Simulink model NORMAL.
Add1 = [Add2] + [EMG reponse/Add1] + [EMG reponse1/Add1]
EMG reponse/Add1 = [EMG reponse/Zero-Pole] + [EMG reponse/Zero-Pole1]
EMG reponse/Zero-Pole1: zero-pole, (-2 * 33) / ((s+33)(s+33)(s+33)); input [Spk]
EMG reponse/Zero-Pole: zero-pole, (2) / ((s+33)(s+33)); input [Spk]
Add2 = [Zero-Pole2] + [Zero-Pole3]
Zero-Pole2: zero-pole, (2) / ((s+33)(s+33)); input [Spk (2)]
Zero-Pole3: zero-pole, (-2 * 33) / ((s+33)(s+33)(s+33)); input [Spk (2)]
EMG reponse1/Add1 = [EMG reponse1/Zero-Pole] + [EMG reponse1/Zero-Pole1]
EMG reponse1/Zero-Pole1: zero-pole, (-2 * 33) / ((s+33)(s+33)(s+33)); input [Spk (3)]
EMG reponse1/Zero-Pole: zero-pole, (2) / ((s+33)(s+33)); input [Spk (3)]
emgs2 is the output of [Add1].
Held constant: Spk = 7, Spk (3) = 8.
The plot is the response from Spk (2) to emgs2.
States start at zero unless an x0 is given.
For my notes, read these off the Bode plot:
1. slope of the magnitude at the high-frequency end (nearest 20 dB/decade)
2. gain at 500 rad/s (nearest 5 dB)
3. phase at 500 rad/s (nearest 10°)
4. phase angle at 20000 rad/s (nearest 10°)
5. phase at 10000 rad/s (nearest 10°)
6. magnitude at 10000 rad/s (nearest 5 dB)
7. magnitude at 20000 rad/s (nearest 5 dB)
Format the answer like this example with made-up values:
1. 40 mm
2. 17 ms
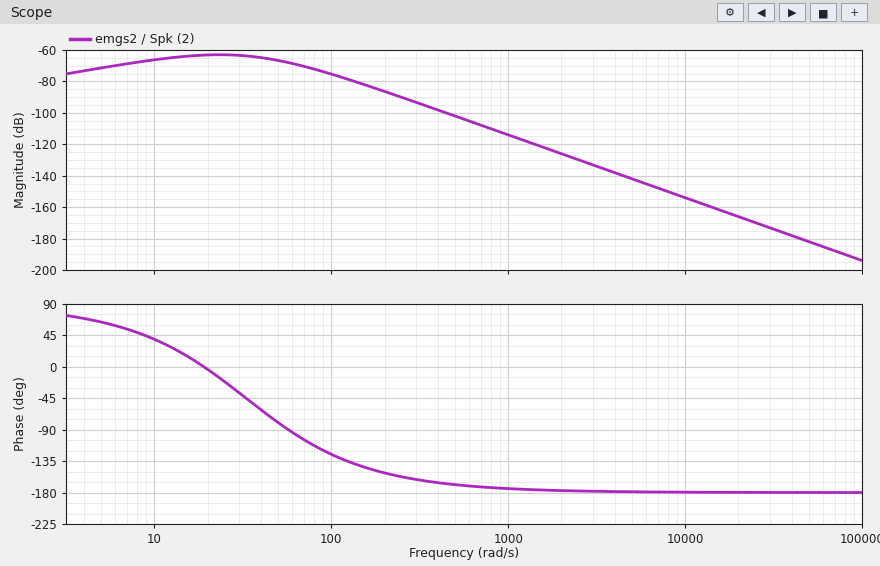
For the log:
1. -40 dB/decade
2. -100 dB
3. -170°
4. -180°
5. -180°
6. -155 dB
7. -165 dB
